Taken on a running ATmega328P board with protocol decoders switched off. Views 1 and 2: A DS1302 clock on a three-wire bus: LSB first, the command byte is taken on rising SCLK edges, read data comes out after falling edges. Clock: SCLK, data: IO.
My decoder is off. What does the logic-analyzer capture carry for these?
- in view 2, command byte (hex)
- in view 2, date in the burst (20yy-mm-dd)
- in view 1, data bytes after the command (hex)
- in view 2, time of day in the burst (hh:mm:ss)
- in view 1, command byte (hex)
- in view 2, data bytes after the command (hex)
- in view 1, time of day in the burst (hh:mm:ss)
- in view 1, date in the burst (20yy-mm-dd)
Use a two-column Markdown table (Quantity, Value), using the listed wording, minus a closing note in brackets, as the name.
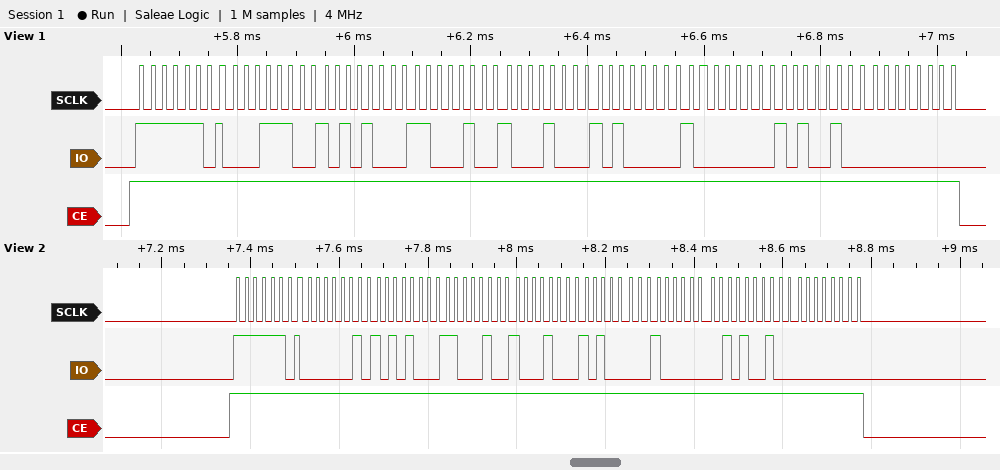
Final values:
| Quantity | Value |
|---|---|
| in view 2, command byte | 0xBF |
| in view 2, date in the burst | 2025-05-11 |
| in view 1, data bytes after the command | 38 15 23 11 05 01 25 00 |
| in view 2, time of day in the burst | 23:15:40 |
| in view 1, command byte | 0xBF |
| in view 2, data bytes after the command | 40 15 23 11 05 01 25 00 |
| in view 1, time of day in the burst | 23:15:38 |
| in view 1, date in the burst | 2025-05-11 |
